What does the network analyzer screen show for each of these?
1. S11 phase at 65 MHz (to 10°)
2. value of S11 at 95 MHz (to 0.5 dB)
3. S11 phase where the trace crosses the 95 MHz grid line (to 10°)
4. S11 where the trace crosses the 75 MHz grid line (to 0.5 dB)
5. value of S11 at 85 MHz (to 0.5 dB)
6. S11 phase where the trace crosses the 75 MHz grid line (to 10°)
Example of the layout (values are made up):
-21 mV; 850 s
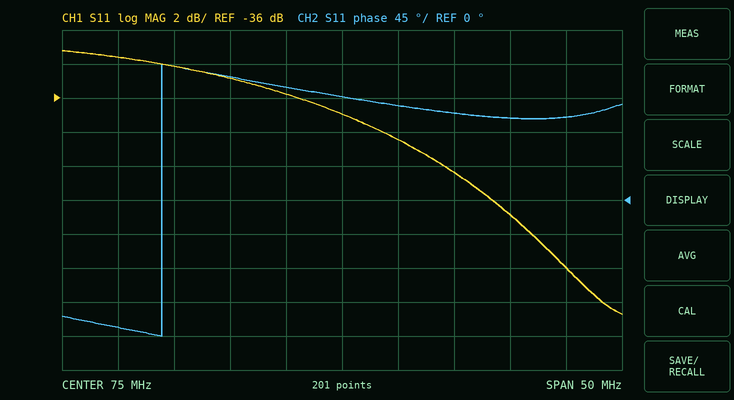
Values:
160°; -46.0 dB; 110°; -37.0 dB; -40.5 dB; 140°
